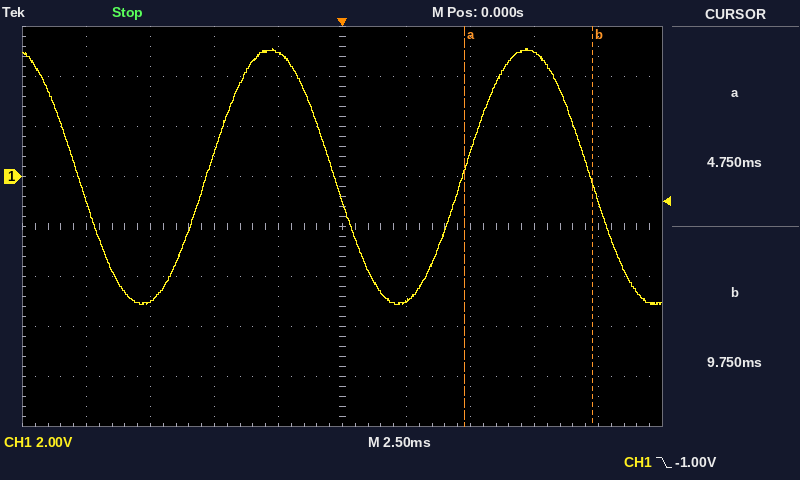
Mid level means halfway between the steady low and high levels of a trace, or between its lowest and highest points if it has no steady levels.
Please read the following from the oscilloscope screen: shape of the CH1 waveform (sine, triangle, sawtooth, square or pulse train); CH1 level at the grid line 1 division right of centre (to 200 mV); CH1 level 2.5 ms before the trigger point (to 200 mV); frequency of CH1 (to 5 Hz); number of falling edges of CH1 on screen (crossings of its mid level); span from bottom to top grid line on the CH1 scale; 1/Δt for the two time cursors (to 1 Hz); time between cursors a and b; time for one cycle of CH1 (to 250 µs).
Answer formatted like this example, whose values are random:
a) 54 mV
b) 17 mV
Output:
a) sine
b) -5.0 V
c) 5.0 V
d) 100 Hz
e) 3
f) 16 V
g) 200 Hz
h) 5.00 ms
i) 10.00 ms
